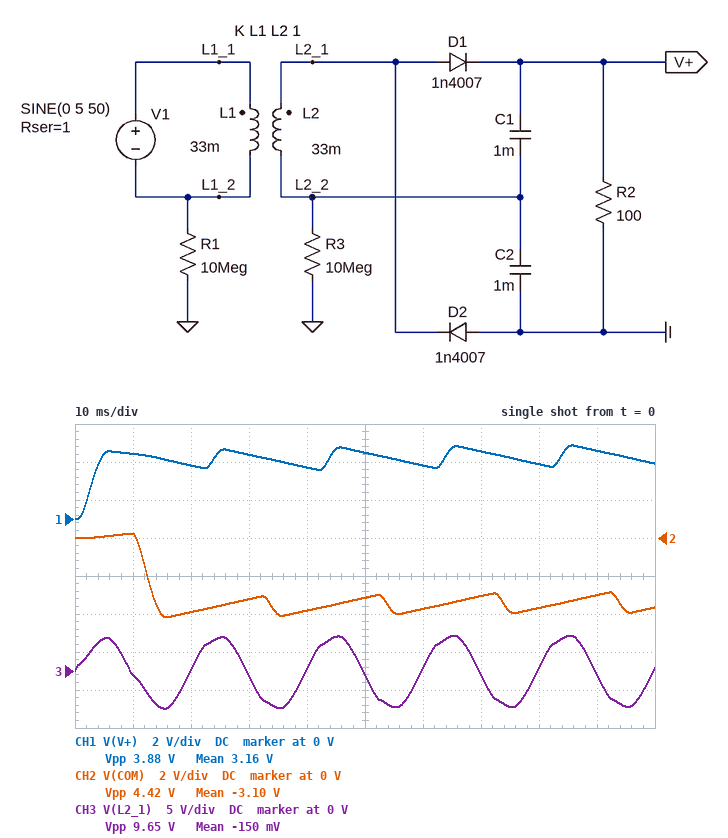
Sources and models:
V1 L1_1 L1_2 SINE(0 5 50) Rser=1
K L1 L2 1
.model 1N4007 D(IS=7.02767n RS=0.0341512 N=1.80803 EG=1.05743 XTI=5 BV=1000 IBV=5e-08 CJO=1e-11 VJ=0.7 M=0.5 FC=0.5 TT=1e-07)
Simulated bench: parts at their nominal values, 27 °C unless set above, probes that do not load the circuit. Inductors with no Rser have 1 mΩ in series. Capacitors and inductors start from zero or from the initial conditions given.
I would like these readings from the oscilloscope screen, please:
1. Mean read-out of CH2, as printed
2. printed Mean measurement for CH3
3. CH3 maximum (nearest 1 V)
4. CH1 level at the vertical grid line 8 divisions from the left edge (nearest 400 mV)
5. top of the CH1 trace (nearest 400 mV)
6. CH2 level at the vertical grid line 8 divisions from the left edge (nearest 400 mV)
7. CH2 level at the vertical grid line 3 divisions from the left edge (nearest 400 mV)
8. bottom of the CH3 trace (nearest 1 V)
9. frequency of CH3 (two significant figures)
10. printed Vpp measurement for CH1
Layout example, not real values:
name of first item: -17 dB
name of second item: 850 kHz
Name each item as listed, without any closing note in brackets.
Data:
Mean read-out of CH2, as printed: -3.10 V
printed Mean measurement for CH3: -150 mV
CH3 maximum: 5 V
CH1 level at the vertical grid line 8 divisions from the left edge: 2.8 V
top of the CH1 trace: 4.0 V
CH2 level at the vertical grid line 8 divisions from the left edge: -3.6 V
CH2 level at the vertical grid line 3 divisions from the left edge: -3.2 V
bottom of the CH3 trace: -5 V
frequency of CH3: 50 Hz
printed Vpp measurement for CH1: 3.88 V
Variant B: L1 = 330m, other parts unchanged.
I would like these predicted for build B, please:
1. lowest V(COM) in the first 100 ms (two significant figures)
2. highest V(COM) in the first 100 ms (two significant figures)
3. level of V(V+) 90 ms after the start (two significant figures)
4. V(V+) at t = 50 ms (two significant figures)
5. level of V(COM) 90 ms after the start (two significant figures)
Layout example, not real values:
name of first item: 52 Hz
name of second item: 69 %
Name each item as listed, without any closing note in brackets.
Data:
lowest V(COM) in the first 100 ms: -850 mV
highest V(COM) in the first 100 ms: 62 mV
level of V(V+) 90 ms after the start: 770 mV
V(V+) at t = 50 ms: 760 mV
level of V(COM) 90 ms after the start: -650 mV
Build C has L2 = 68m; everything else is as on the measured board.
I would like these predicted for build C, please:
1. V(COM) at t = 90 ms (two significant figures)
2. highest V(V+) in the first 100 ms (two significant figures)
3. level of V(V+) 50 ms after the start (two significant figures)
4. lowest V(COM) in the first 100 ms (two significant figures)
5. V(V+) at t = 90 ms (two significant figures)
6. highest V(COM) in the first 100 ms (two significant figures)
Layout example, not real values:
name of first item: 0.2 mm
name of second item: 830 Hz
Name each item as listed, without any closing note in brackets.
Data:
V(COM) at t = 90 ms: -4.3 V
highest V(V+) in the first 100 ms: 5.4 V
level of V(V+) 50 ms after the start: 4.9 V
lowest V(COM) in the first 100 ms: -5.8 V
V(V+) at t = 90 ms: 5.1 V
highest V(COM) in the first 100 ms: 300 mV
